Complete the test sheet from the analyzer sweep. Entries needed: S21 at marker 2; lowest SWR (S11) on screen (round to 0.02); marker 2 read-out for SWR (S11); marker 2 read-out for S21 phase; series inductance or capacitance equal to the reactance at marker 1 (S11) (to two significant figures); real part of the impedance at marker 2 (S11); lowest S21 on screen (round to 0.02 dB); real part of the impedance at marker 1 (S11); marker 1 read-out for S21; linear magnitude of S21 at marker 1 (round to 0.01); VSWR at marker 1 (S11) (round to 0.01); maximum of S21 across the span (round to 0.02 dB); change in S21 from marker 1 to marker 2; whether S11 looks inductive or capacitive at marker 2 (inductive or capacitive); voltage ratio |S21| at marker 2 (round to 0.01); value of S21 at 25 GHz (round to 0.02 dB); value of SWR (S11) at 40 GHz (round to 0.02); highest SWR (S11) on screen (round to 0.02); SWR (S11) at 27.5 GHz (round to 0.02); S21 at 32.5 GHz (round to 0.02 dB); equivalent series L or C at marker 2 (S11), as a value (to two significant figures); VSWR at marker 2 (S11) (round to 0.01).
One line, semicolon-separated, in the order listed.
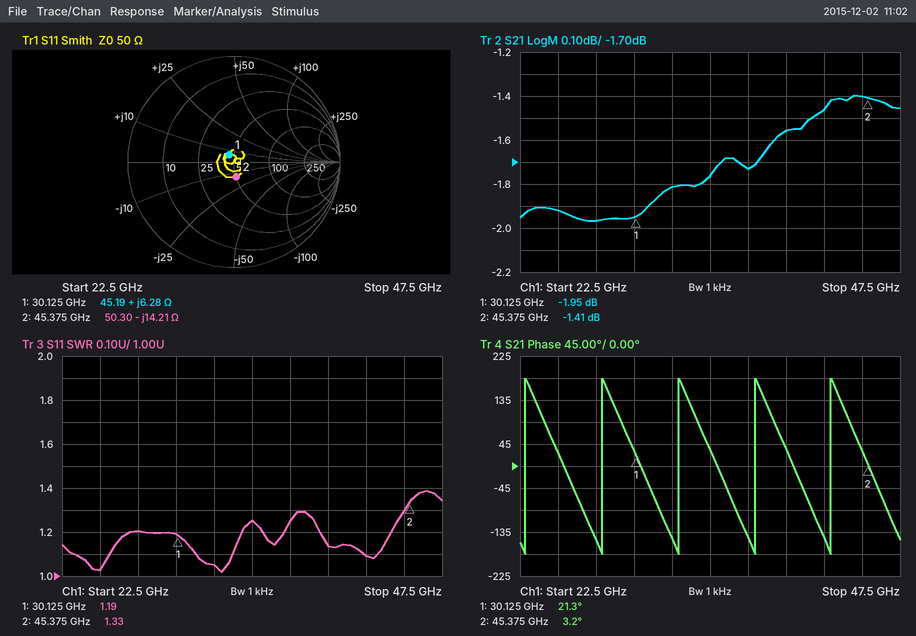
-1.41 dB; 1.02; 1.33; 3.2°; 33 pH; 50.30 Ω; -1.96 dB; 45.19 Ω; -1.95 dB; 0.80; 1.18; -1.40 dB; 0.54 dB; capacitive; 0.85; -1.92 dB; 1.14; 1.38; 1.20; -1.82 dB; 250 fF; 1.33
